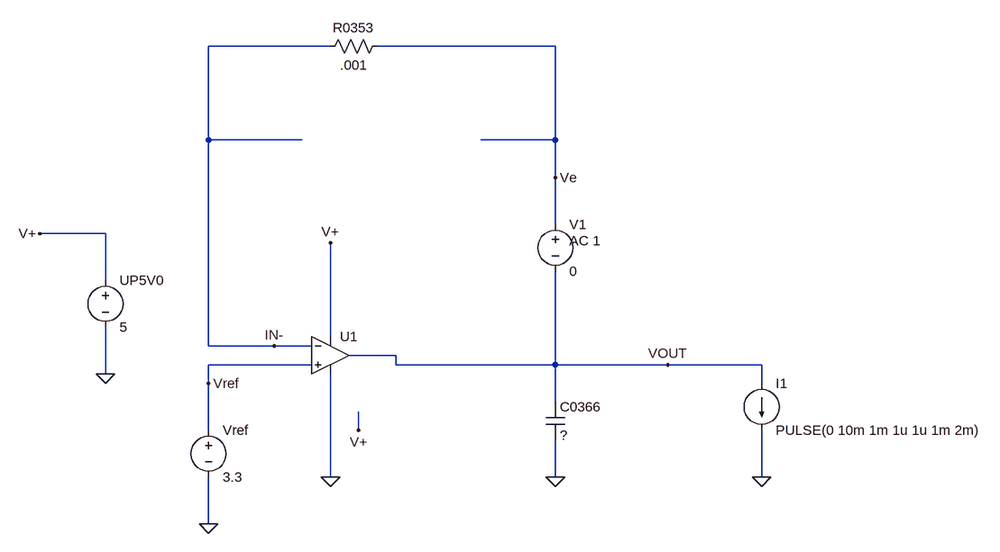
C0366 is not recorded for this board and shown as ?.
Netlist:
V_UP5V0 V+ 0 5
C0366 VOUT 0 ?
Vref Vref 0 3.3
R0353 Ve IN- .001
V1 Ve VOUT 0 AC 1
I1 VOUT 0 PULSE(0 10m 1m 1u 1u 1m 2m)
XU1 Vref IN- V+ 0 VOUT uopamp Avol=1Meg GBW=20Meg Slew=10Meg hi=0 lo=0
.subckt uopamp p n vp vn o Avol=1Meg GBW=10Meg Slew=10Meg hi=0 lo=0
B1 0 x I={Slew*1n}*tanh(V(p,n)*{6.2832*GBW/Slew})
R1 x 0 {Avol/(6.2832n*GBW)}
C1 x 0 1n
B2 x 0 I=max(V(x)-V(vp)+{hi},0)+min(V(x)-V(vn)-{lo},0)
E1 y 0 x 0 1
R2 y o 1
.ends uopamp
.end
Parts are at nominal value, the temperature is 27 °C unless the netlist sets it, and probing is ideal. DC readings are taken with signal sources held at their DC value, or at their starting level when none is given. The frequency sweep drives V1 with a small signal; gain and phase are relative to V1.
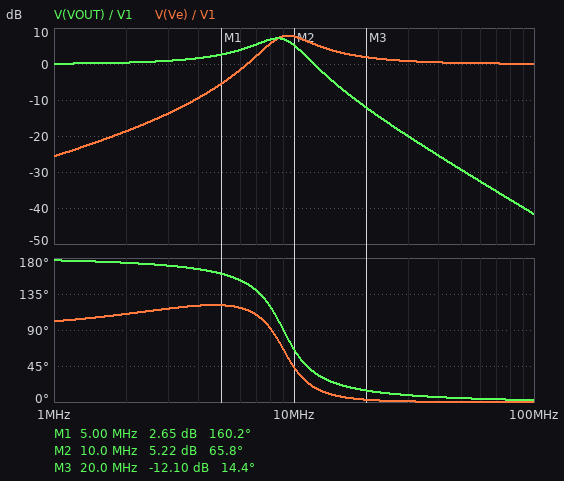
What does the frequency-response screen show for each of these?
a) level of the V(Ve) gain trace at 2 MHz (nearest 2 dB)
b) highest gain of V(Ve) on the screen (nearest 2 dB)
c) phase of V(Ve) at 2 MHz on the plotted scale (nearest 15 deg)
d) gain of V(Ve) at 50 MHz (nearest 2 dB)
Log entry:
-18 dB
8 dB
105 deg
0 dB
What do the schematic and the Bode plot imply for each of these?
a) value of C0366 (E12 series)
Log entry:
39 nF
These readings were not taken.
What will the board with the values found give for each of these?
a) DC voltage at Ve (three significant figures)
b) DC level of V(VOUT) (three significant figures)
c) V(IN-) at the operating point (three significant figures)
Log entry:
3.30 V
3.30 V
3.30 V
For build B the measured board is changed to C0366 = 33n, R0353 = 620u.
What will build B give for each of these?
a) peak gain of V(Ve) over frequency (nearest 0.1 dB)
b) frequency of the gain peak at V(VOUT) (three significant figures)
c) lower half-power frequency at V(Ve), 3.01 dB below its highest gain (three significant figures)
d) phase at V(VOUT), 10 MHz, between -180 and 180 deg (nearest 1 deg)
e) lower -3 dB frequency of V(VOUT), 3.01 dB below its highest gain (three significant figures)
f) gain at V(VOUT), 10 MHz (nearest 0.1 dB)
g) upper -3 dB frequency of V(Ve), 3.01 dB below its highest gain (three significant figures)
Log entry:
7.3 dB
9.21 MHz
8.30 MHz
86 deg
6.24 MHz
6.0 dB
14.7 MHz
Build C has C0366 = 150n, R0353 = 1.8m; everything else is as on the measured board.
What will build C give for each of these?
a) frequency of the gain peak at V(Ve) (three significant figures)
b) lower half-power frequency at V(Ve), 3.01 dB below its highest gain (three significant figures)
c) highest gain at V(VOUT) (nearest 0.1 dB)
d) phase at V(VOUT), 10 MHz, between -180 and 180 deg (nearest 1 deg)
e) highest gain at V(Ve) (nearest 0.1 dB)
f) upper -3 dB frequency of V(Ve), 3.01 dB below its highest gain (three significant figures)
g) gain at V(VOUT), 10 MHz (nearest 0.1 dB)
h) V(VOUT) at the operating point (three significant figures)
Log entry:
4.67 MHz
4.20 MHz
12.8 dB
8 deg
13.0 dB
5.33 MHz
-11.5 dB
3.30 V
